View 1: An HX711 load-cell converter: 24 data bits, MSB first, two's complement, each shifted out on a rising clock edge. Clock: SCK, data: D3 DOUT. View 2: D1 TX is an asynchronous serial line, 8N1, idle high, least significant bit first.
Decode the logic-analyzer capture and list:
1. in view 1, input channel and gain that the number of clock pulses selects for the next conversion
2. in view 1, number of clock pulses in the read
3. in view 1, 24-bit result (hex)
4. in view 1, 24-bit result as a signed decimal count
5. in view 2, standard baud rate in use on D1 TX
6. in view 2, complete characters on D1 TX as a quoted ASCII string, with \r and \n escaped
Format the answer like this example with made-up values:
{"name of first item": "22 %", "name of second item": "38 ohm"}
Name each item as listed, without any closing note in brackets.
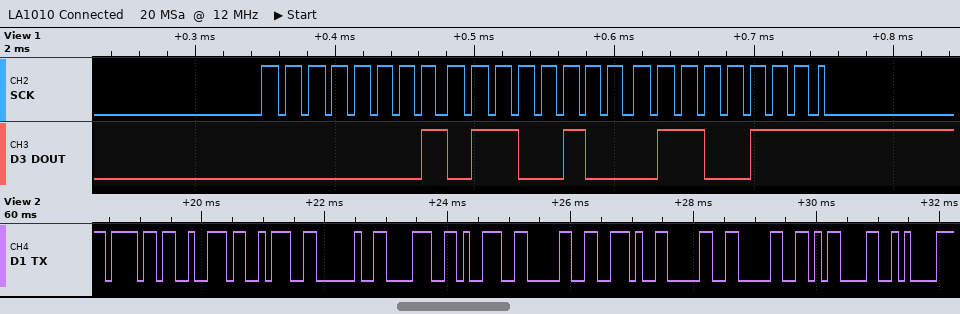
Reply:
{"in view 1, input channel and gain that the number of clock pulses selects for the next conversion": "channel A, gain 128", "in view 1, number of clock pulses in the read": "25", "in view 1, 24-bit result": "0x016467", "in view 1, 24-bit result as a signed decimal count": "91239", "in view 2, standard baud rate in use on D1 TX": "9600 baud", "in view 2, complete characters on D1 TX as a quoted ASCII string, with \\r and \\n escaped": "\"or: 890.00\\r\\n\""}
